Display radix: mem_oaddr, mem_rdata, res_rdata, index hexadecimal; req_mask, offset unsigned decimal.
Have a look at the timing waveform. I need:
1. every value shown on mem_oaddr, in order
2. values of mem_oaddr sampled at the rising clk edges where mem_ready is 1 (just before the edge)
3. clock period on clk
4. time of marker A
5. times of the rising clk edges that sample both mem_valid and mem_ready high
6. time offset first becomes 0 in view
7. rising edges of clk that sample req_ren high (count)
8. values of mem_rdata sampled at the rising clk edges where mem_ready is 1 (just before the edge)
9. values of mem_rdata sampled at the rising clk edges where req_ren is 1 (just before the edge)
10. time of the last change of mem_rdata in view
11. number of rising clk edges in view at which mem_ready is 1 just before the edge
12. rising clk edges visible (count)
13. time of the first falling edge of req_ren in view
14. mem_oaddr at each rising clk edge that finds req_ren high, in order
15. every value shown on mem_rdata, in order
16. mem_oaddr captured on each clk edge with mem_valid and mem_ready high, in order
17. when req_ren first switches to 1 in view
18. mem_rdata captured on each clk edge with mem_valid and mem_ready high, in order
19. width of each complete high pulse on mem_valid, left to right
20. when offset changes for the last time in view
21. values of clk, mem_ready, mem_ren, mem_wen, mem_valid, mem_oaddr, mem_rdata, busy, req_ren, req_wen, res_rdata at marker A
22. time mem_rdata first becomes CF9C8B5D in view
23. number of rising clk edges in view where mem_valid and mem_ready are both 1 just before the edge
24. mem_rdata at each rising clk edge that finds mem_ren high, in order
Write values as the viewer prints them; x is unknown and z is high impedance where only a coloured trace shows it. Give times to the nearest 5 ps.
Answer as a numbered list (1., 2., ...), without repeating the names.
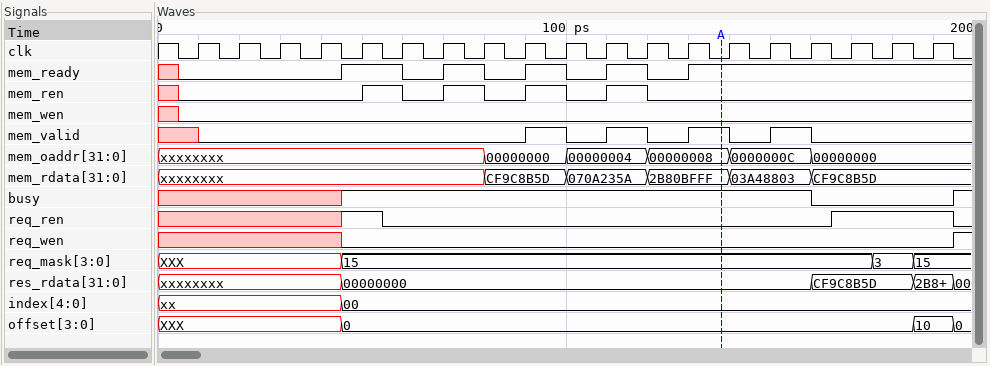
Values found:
1. xxxxxxxx, 00000000, 00000004, 00000008, 0000000C, 00000000
2. xxxxxxxx, xxxxxxxx, xxxxxxxx, 00000000, 00000004, 00000008, 0000000C, 0000000C, 00000000, 00000000, 00000000
3. 10 ps
4. 140 ps
5. 100 ps, 120 ps, 140 ps, 160 ps
6. 45 ps
7. 4
8. xxxxxxxx, xxxxxxxx, xxxxxxxx, CF9C8B5D, 070A235A, 2B80BFFF, 03A48803, 03A48803, CF9C8B5D, CF9C8B5D, CF9C8B5D
9. xxxxxxxx, CF9C8B5D, CF9C8B5D, CF9C8B5D
10. 160 ps
11. 11
12. 19
13. 55 ps
14. xxxxxxxx, 00000000, 00000000, 00000000
15. xxxxxxxx, CF9C8B5D, 070A235A, 2B80BFFF, 03A48803, CF9C8B5D
16. 00000000, 00000004, 00000008, 0000000C
17. 45 ps
18. CF9C8B5D, 070A235A, 2B80BFFF, 03A48803
19. 10 ps, 10 ps, 10 ps, 10 ps
20. 195 ps
21. clk=0, mem_ready=1, mem_ren=0, mem_wen=0, mem_valid=1, mem_oaddr=00000008, mem_rdata=2B80BFFF, busy=1, req_ren=0, req_wen=0, res_rdata=00000000
22. 80 ps
23. 4
24. xxxxxxxx, xxxxxxxx, CF9C8B5D, 070A235A
